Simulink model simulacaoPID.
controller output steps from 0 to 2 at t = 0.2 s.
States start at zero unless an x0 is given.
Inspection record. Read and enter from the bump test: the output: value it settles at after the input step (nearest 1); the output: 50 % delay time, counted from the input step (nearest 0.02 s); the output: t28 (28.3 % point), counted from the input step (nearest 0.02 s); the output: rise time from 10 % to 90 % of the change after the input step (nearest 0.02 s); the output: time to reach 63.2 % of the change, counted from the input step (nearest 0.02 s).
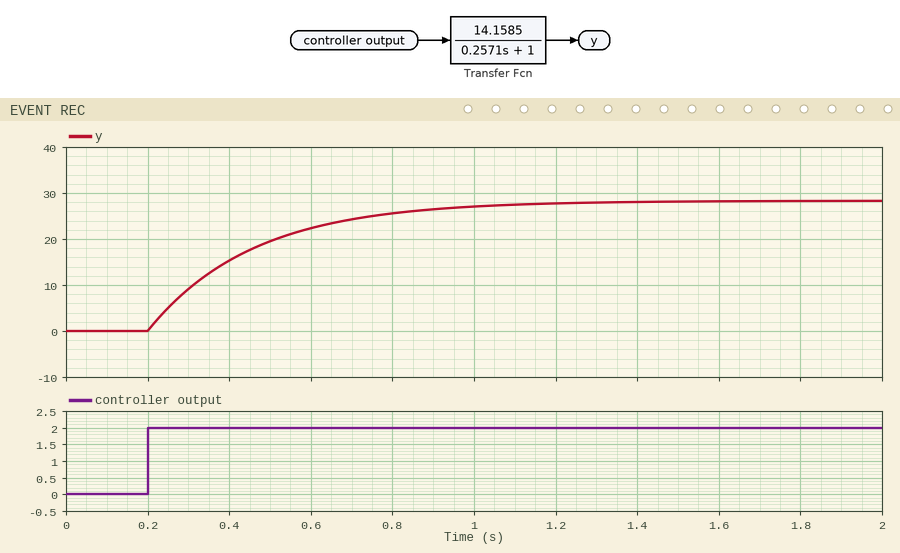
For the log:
28
0.18 s
0.08 s
0.56 s
0.26 s
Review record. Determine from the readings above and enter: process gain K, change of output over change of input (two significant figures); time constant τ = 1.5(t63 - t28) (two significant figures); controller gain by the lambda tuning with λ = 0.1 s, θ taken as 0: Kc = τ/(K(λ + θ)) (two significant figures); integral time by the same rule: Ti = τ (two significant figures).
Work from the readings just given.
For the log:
14
0.27 s
0.19
0.27 s
